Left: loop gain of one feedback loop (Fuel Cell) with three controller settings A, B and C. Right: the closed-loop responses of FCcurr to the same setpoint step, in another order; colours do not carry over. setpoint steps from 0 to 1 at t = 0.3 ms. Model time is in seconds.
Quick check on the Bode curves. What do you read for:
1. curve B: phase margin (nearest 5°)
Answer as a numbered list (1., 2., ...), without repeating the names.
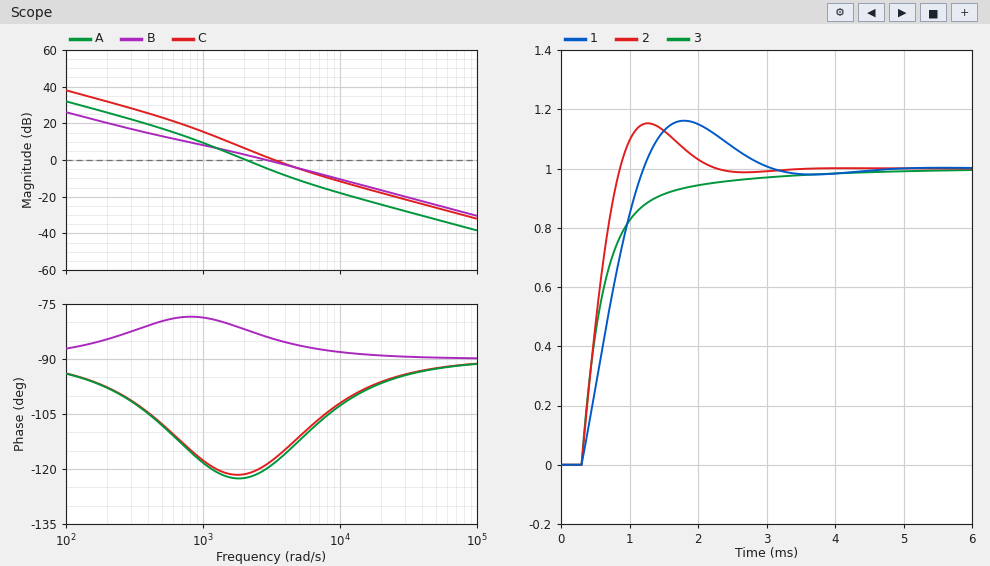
1. 95°
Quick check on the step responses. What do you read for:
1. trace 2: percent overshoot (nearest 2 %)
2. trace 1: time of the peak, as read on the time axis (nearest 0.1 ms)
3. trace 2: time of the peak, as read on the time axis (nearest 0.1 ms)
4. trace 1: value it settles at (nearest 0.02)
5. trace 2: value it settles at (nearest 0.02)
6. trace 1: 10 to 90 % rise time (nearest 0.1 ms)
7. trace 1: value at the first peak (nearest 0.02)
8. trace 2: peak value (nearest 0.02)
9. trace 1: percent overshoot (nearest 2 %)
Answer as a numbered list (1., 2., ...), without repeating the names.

1. 16 %
2. 1.8 ms
3. 1.3 ms
4. 1.00
5. 1.00
6. 0.7 ms
7. 1.16
8. 1.16
9. 16 %
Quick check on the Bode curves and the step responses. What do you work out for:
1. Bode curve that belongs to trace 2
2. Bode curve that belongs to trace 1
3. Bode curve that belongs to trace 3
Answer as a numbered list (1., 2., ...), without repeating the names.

1. C
2. A
3. B
